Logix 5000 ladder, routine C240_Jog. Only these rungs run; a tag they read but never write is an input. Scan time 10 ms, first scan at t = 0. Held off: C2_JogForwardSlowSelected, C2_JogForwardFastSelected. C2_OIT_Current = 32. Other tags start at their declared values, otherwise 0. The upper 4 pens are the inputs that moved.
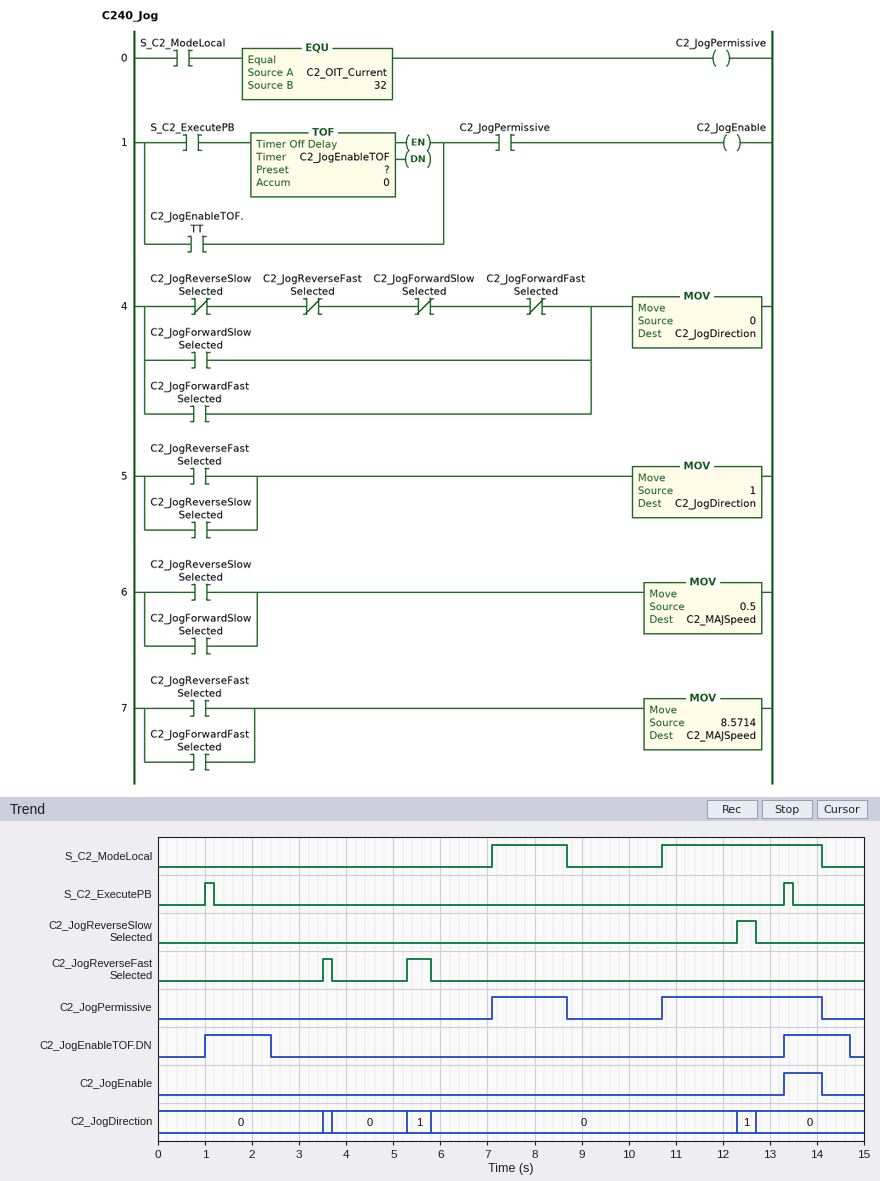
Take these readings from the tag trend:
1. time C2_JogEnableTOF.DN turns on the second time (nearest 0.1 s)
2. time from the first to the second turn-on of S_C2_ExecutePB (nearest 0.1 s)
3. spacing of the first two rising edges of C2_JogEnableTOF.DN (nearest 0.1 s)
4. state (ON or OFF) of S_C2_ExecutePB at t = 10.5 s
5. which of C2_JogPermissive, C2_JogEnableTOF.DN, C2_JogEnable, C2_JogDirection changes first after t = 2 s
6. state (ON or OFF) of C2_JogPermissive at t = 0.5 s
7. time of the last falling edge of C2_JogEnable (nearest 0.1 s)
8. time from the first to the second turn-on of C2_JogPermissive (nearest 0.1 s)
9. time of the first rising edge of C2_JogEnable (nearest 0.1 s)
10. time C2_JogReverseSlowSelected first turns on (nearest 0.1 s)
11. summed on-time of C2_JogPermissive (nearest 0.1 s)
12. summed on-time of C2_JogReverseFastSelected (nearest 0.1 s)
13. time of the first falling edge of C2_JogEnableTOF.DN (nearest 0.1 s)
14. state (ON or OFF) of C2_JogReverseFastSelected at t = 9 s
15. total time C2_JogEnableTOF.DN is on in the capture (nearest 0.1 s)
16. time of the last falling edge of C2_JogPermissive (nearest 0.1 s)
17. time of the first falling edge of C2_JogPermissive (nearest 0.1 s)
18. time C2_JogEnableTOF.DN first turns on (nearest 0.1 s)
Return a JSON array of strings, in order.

["13.3 s", "12.3 s", "12.3 s", "OFF", "C2_JogEnableTOF.DN", "OFF", "14.1 s", "3.6 s", "13.3 s", "12.3 s", "5.0 s", "0.7 s", "2.4 s", "OFF", "2.8 s", "14.1 s", "8.7 s", "1.0 s"]
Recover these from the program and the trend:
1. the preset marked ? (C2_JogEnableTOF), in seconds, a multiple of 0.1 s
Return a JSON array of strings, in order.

["1.2 s"]
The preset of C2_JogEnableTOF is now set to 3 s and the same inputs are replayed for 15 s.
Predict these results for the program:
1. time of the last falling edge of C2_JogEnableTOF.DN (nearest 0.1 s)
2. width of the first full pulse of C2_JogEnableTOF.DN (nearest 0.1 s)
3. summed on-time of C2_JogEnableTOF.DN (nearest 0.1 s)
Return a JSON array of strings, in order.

["4.2 s", "3.2 s", "4.9 s"]
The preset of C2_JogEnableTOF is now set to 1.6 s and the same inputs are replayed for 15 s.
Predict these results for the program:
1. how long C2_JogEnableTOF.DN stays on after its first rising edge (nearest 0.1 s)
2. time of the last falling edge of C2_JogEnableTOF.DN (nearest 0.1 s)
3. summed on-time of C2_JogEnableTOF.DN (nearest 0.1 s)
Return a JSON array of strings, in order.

["1.8 s", "2.8 s", "3.5 s"]
